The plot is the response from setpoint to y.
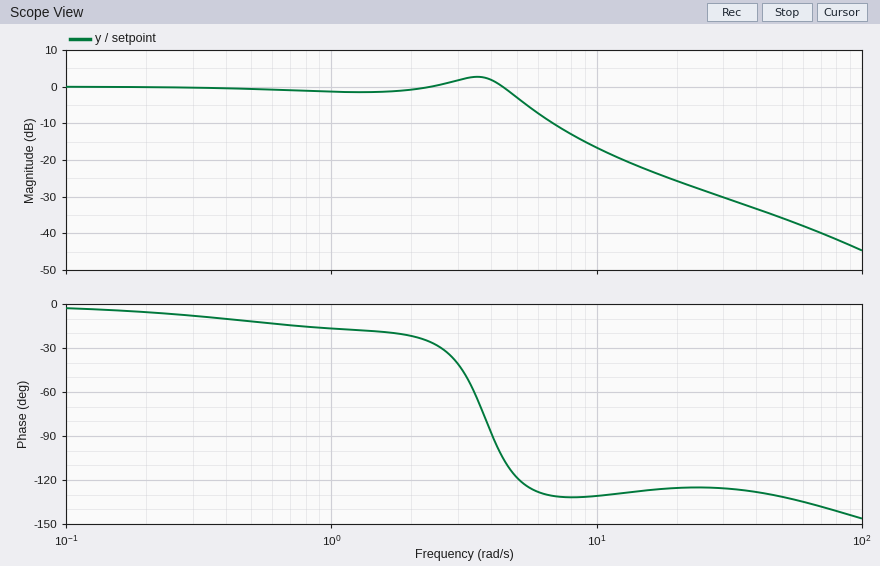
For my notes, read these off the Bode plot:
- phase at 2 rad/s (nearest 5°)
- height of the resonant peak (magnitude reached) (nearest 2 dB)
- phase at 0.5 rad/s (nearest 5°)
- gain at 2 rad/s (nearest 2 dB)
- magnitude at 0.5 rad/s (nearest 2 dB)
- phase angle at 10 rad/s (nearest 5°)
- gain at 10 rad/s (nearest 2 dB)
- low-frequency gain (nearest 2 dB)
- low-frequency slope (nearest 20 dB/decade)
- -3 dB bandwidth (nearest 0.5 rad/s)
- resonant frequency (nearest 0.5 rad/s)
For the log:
-20°
2 dB
-10°
0 dB
0 dB
-130°
-16 dB
0 dB
0 dB/decade
5.0 rad/s
3.5 rad/s
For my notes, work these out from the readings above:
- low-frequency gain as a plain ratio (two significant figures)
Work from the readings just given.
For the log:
1.0
